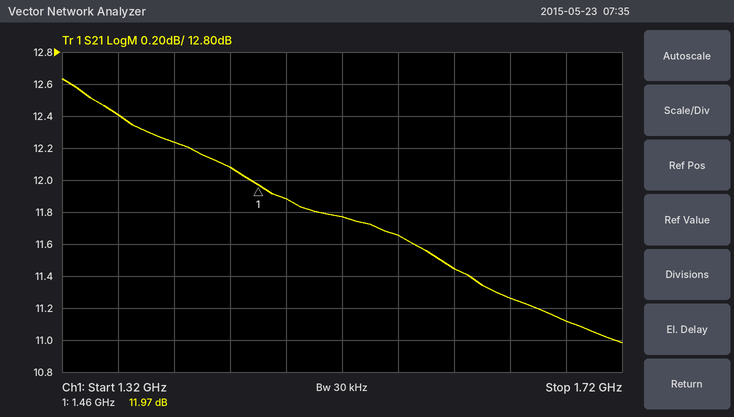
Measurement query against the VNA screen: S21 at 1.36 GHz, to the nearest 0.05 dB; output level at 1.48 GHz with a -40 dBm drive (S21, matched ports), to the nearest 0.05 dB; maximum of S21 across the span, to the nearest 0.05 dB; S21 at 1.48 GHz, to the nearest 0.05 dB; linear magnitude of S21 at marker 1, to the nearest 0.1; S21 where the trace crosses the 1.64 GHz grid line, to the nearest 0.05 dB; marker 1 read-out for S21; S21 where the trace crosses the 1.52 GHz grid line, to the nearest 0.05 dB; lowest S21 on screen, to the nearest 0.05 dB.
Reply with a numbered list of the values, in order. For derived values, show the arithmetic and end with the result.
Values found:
1. 12.40 dB
2. -40 dBm + (11.90 dB) = -28.10 dBm
3. 12.65 dB
4. 11.90 dB
5. 10^(11.97/20) ≈ 4.0
6. 11.25 dB
7. 11.97 dB
8. 11.75 dB
9. 11.00 dB
